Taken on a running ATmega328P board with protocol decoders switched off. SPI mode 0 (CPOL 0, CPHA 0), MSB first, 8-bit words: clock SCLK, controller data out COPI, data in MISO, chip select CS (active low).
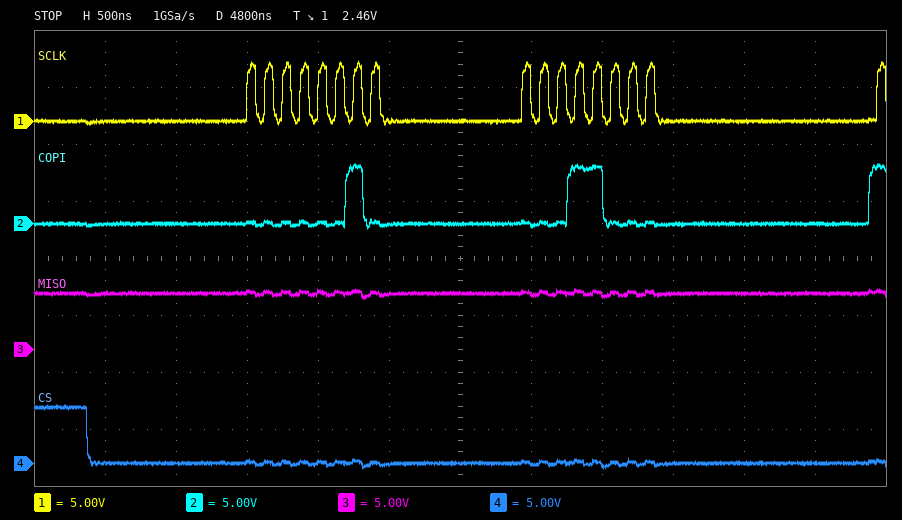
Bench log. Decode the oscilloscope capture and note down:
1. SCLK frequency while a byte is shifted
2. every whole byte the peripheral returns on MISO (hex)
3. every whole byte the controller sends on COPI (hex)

8 MHz
FF FF
02 18
